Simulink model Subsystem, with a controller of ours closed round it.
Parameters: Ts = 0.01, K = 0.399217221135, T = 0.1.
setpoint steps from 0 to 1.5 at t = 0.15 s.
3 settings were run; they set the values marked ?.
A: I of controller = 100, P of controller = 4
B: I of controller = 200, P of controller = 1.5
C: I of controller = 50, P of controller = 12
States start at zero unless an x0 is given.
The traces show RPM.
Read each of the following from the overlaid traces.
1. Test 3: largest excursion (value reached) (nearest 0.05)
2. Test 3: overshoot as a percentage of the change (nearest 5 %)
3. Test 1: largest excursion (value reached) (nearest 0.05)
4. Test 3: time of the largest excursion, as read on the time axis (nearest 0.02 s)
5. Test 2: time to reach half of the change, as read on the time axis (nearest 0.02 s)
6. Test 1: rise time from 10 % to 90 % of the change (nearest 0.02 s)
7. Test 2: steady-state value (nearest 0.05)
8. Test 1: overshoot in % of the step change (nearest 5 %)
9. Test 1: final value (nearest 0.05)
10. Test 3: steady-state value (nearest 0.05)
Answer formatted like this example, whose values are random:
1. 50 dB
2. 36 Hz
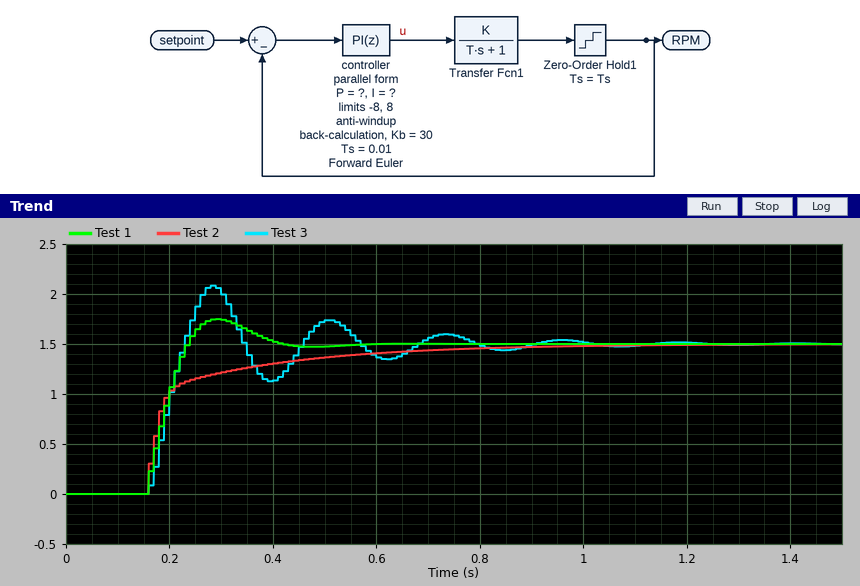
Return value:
1. 2.10
2. 40 %
3. 1.75
4. 0.28 s
5. 0.18 s
6. 0.06 s
7. 1.50
8. 15 %
9. 1.50
10. 1.50
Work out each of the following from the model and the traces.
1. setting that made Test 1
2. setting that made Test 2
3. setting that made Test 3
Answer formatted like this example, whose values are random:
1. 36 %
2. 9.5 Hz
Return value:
1. A
2. C
3. B
